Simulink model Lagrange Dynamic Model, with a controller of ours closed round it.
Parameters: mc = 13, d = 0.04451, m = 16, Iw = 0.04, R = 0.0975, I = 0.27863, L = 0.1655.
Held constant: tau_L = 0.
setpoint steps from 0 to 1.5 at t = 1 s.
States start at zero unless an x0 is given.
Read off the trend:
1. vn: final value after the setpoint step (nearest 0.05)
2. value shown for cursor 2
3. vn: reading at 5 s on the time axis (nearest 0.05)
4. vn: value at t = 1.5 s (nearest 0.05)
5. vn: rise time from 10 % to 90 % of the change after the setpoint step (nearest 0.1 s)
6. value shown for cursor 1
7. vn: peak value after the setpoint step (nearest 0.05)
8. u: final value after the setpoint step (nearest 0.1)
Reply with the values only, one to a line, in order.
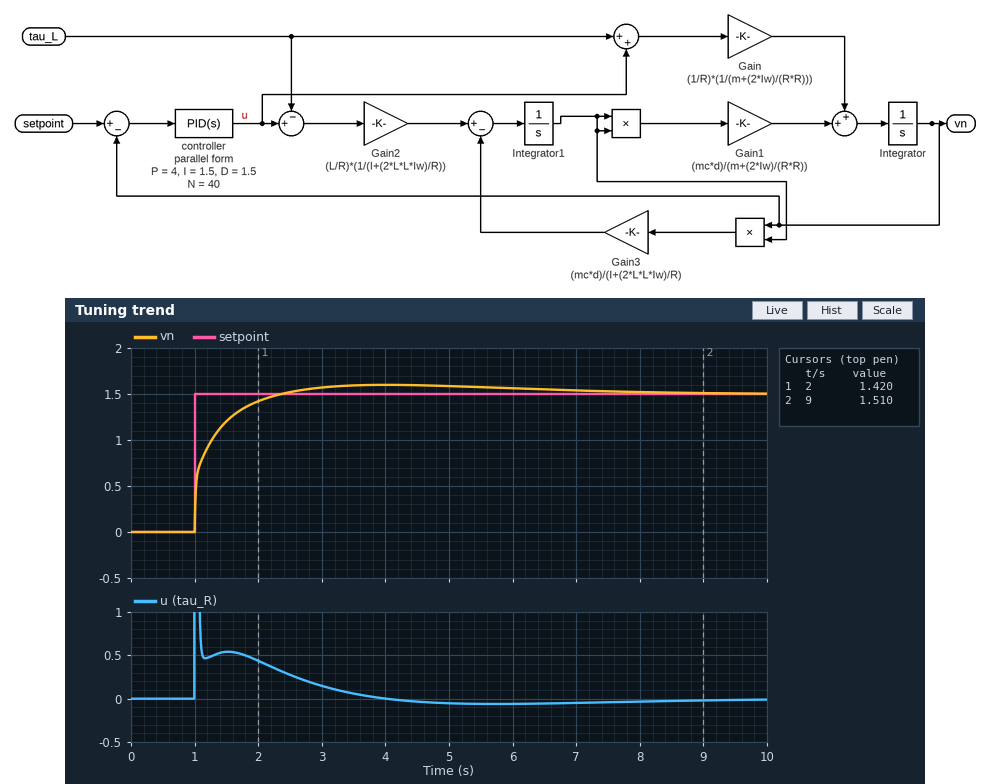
1.50
1.510
1.60
1.20
0.8 s
1.420
1.60
0.0
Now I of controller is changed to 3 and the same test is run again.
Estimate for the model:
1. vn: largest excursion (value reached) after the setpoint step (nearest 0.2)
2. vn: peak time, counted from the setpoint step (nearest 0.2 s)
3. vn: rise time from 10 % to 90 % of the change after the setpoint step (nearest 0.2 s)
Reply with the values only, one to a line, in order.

1.6
2.2 s
0.6 s
